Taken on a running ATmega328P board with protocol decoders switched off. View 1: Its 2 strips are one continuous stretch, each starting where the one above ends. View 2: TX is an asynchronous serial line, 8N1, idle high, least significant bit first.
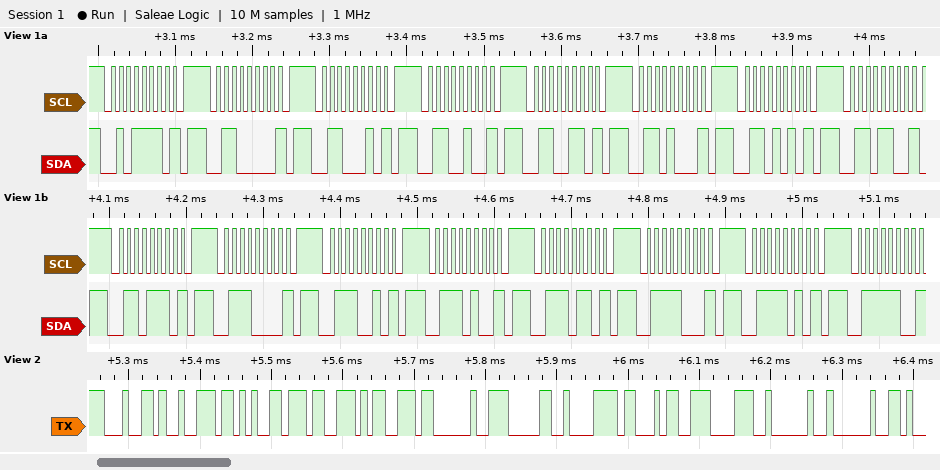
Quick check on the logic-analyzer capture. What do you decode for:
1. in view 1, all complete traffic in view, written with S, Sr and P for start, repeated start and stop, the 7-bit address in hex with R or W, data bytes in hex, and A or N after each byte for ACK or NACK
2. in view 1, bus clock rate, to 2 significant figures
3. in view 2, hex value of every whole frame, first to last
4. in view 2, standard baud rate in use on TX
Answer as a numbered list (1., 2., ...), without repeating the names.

1. S 2FW N P S 30W N P S 31W N P S 32W N P S 33W N P S 34W N P S 35W N P S 36W N P S 37W N P S 38W N P S 39W N P S 3AW N P S 3BW N P S 3CW N P S 3DW N P S 3EW N
2. 100 kHz
3. 64 72 65 73 73 20 30 78 34 38 20 20
4. 115200 baud
